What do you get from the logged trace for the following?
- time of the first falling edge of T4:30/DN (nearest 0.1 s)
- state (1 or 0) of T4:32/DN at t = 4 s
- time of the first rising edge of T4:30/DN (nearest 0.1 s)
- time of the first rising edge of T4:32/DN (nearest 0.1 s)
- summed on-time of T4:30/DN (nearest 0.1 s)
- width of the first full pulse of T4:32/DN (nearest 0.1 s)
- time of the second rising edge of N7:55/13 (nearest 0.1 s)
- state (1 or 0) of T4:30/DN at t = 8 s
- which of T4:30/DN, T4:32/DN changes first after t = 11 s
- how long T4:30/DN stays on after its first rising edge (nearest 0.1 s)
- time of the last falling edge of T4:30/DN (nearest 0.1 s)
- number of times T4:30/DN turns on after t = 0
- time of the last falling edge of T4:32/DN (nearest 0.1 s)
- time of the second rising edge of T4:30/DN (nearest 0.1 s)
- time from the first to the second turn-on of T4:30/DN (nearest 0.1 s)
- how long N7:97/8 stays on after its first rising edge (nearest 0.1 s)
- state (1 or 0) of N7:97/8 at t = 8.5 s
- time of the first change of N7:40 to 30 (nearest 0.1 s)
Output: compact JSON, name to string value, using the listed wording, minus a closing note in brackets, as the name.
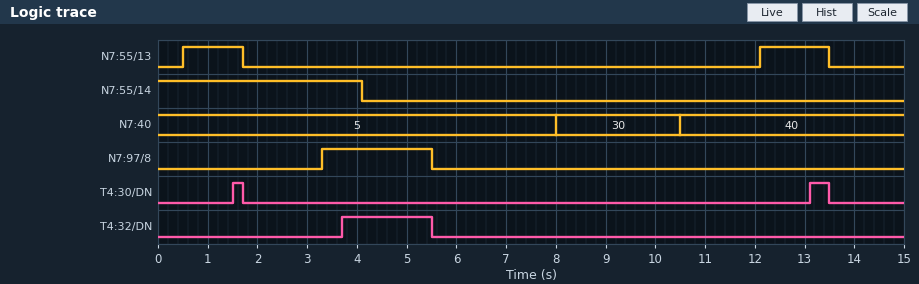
{"time of the first falling edge of T4:30/DN": "1.7 s", "state (1 or 0) of T4:32/DN at t = 4 s": "1", "time of the first rising edge of T4:30/DN": "1.5 s", "time of the first rising edge of T4:32/DN": "3.7 s", "summed on-time of T4:30/DN": "0.6 s", "width of the first full pulse of T4:32/DN": "1.8 s", "time of the second rising edge of N7:55/13": "12.1 s", "state (1 or 0) of T4:30/DN at t = 8 s": "0", "which of T4:30/DN, T4:32/DN changes first after t = 11 s": "T4:30/DN", "how long T4:30/DN stays on after its first rising edge": "0.2 s", "time of the last falling edge of T4:30/DN": "13.5 s", "number of times T4:30/DN turns on after t = 0": "2", "time of the last falling edge of T4:32/DN": "5.5 s", "time of the second rising edge of T4:30/DN": "13.1 s", "time from the first to the second turn-on of T4:30/DN": "11.6 s", "how long N7:97/8 stays on after its first rising edge": "2.2 s", "state (1 or 0) of N7:97/8 at t = 8.5 s": "0", "time of the first change of N7:40 to 30": "8.0 s"}
